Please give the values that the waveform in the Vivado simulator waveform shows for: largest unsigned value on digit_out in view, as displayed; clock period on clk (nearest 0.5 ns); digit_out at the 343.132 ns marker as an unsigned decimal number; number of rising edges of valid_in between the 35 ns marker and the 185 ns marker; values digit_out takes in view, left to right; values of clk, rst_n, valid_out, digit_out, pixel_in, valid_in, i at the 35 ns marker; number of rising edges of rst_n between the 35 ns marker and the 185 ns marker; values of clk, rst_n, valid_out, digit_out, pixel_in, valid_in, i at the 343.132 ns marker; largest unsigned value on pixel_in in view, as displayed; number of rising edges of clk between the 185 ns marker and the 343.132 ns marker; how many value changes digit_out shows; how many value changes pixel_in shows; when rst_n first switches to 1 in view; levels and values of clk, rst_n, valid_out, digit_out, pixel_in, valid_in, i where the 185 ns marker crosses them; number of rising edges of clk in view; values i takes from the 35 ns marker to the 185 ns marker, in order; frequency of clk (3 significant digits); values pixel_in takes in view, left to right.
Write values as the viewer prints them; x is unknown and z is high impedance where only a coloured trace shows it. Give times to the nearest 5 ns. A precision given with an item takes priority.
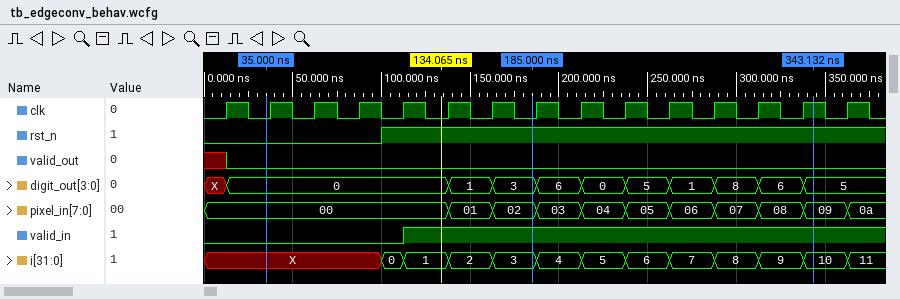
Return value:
8
25 ns
5
1
X, 0, 1, 3, 6, 0, 5, 1, 8, 6, 5
clk=0, rst_n=0, valid_out=0, digit_out=0, pixel_in=00, valid_in=0, i=X
1
clk=1, rst_n=1, valid_out=0, digit_out=5, pixel_in=09, valid_in=1, i=10
0a
7
10
10
100 ns
clk=0, rst_n=1, valid_out=0, digit_out=3, pixel_in=02, valid_in=1, i=3
15
X, 0, 1, 2, 3
40.0 MHz
00, 01, 02, 03, 04, 05, 06, 07, 08, 09, 0a
